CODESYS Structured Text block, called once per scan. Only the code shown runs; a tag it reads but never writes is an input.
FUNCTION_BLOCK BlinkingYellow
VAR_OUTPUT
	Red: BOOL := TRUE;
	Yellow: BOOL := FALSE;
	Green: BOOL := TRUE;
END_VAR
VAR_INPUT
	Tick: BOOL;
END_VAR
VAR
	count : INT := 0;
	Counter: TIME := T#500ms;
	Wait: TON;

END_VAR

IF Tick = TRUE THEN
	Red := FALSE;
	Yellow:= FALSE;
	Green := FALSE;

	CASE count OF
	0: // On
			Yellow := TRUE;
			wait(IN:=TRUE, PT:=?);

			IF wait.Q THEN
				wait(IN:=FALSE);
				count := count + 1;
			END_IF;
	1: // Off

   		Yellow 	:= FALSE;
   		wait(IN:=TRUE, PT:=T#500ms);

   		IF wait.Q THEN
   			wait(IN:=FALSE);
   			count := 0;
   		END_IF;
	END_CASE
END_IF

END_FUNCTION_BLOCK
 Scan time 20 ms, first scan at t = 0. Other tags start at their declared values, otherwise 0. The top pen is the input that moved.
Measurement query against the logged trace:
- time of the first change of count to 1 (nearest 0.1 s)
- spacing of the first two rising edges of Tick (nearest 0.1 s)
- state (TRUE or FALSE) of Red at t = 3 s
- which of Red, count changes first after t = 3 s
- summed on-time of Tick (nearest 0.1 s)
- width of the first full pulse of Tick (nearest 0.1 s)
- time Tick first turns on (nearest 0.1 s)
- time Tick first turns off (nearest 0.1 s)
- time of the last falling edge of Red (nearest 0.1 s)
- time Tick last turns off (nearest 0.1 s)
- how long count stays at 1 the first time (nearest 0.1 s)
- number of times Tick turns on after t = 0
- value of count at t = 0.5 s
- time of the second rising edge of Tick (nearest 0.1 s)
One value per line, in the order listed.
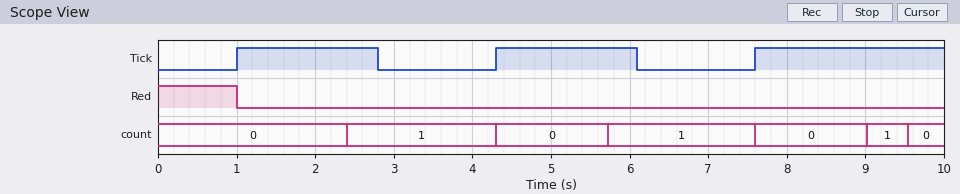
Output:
2.4 s
3.3 s
FALSE
count
6.0 s
1.8 s
1.0 s
2.8 s
1.0 s
6.1 s
1.9 s
3
0
4.3 s
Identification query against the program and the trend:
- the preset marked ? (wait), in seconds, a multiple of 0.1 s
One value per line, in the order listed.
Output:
1.4 s
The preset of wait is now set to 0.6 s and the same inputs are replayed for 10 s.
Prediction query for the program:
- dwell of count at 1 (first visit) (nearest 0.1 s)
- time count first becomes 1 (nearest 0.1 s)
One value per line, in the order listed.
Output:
0.5 s
1.6 s
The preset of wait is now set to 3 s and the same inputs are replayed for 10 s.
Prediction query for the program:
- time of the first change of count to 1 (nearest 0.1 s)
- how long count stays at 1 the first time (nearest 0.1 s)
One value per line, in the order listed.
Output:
4.3 s
0.5 s
